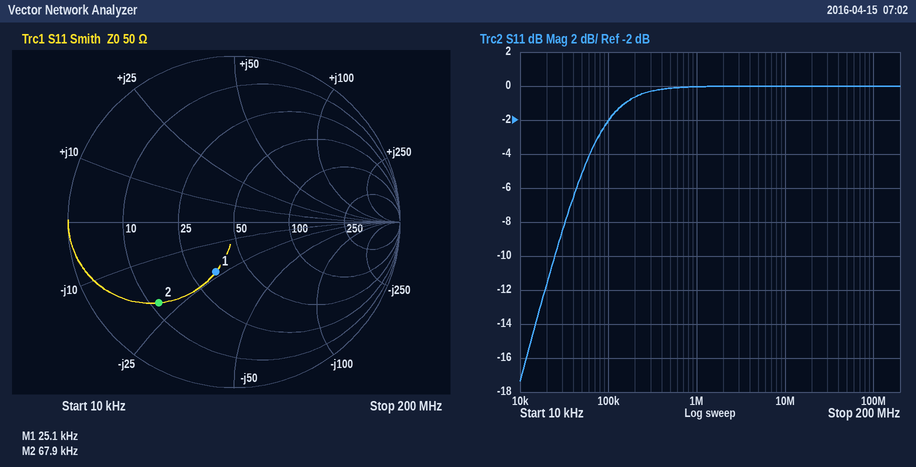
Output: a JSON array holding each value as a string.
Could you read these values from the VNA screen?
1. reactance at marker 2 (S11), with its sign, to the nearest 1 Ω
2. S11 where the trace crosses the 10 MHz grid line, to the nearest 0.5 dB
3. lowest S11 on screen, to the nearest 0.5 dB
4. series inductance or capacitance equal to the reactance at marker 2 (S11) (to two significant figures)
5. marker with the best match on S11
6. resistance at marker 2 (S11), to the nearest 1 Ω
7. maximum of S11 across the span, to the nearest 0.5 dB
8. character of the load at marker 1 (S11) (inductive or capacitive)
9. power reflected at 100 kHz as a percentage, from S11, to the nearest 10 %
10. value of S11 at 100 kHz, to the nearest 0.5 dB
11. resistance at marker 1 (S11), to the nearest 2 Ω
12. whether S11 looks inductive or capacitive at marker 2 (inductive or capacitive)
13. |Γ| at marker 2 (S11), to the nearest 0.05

["-21 Ω", "0.0 dB", "-17.5 dB", "110 nF", "marker 1", "12 Ω", "0.0 dB", "capacitive", "60 %", "-2.0 dB", "34 Ω", "capacitive", "0.65"]
